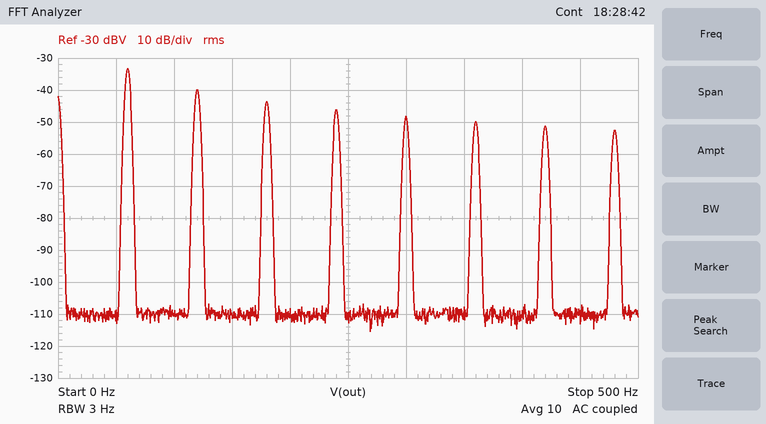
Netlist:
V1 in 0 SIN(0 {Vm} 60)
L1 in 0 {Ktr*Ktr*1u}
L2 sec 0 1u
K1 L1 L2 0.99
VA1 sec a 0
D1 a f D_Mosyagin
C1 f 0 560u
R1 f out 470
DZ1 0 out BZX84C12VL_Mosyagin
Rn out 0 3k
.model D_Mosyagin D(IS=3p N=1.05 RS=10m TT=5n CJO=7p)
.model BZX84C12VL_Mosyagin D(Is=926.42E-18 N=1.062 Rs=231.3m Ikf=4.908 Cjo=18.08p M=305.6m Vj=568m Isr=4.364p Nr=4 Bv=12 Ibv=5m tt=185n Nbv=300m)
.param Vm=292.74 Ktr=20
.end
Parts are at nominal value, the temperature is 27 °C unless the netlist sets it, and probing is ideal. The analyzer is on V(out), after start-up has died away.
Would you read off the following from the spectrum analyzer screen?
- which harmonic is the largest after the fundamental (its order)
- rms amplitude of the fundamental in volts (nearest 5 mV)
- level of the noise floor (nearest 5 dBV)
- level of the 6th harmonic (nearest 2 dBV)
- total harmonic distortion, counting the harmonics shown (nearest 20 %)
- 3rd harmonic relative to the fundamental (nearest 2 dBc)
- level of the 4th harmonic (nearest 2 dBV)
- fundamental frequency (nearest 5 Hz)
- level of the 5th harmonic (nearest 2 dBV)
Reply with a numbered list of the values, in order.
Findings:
1. 2
2. 20 mV
3. -110 dBV
4. -50 dBV
5. 60 %
6. -10 dBc
7. -46 dBV
8. 60 Hz
9. -48 dBV
